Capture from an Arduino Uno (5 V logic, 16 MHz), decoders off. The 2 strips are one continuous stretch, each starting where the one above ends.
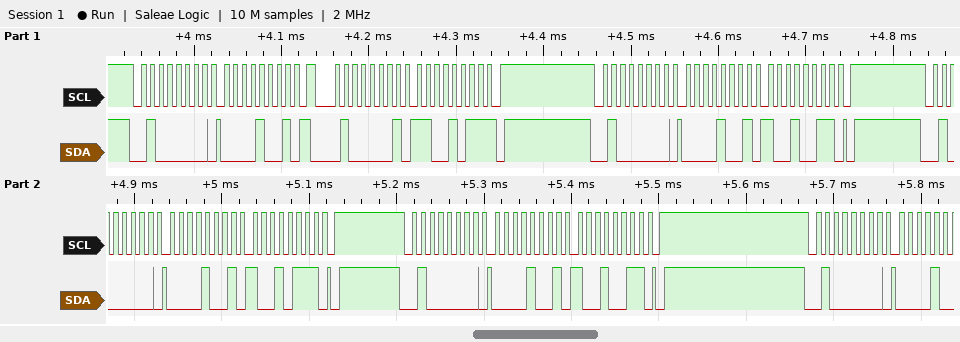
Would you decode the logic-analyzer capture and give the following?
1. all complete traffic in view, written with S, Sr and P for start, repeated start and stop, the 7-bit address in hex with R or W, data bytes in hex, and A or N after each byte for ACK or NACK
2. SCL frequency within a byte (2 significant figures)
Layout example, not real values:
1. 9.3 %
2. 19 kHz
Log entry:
1. S 20W A 09 A Sr 20R A CB N P S 20W A 09 A 93 A P S 20W A 09 A 97 A P S 20W A 09 A 93 A P S 20W A
2. 100 kHz
